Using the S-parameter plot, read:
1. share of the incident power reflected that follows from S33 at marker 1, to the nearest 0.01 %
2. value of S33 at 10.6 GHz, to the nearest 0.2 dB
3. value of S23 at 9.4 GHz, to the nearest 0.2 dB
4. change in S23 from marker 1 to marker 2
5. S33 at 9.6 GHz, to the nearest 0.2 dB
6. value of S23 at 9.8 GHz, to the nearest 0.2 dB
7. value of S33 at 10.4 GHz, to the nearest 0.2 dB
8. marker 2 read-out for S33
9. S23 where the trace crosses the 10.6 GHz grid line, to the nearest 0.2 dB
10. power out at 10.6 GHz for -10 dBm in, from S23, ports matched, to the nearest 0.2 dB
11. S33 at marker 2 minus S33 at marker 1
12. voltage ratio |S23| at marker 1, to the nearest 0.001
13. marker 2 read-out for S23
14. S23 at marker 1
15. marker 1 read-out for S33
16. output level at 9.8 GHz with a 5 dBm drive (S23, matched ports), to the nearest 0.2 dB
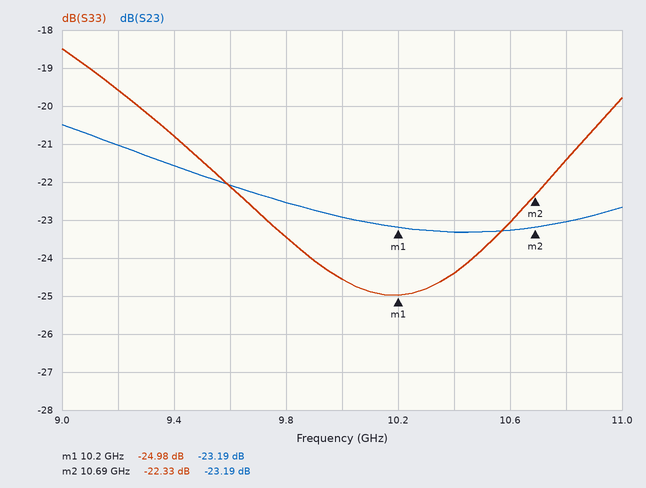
0.32 %
-23.0 dB
-21.6 dB
0.00 dB
-22.2 dB
-22.6 dB
-24.4 dB
-22.33 dB
-23.2 dB
-33.2 dBm
2.65 dB
0.069
-23.19 dB
-23.19 dB
-24.98 dB
-17.6 dBm
